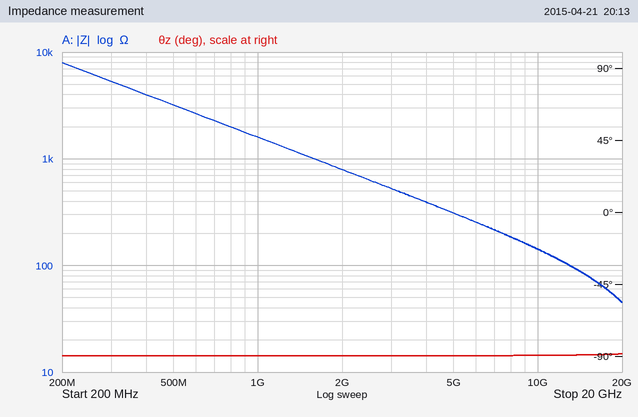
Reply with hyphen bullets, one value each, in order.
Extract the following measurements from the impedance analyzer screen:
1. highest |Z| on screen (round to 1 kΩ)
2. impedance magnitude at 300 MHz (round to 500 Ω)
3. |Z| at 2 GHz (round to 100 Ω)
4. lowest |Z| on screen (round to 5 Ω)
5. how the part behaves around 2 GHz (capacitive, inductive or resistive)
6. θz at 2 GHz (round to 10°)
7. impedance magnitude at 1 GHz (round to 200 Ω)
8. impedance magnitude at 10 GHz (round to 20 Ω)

- 8 kΩ
- 5.5 kΩ
- 800 Ω
- 45 Ω
- capacitive
- -90°
- 1.6 kΩ
- 140 Ω
